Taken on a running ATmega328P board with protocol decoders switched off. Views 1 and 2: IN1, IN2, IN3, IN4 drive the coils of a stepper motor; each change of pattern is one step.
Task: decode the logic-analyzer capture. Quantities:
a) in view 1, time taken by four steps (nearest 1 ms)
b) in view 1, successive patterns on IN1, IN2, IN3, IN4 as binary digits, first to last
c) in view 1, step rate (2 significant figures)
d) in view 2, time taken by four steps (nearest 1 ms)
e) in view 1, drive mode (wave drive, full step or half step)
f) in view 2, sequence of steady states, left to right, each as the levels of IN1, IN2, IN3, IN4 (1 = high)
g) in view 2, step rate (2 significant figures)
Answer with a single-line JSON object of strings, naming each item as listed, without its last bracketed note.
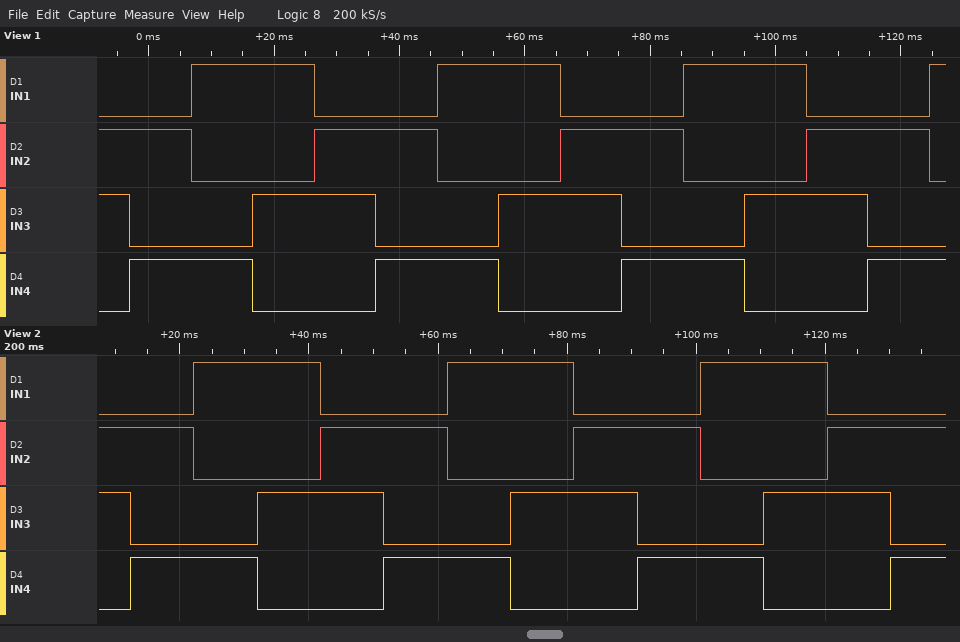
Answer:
{"in view 1, time taken by four steps": "39 ms", "in view 1, successive patterns on IN1, IN2, IN3, IN4 as binary digits, first to last": "0110 0101 1001 1010 0110 0101 1001 1010 0110 0101 1001 1010 0110 0101 1001", "in view 1, step rate": "100 steps/s", "in view 2, time taken by four steps": "39 ms", "in view 1, drive mode": "full step", "in view 2, sequence of steady states, left to right, each as the levels of IN1, IN2, IN3, IN4": "0110 0101 1001 1010 0110 0101 1001 1010 0110 0101 1001 1010 0110 0101", "in view 2, step rate": "100 steps/s"}
